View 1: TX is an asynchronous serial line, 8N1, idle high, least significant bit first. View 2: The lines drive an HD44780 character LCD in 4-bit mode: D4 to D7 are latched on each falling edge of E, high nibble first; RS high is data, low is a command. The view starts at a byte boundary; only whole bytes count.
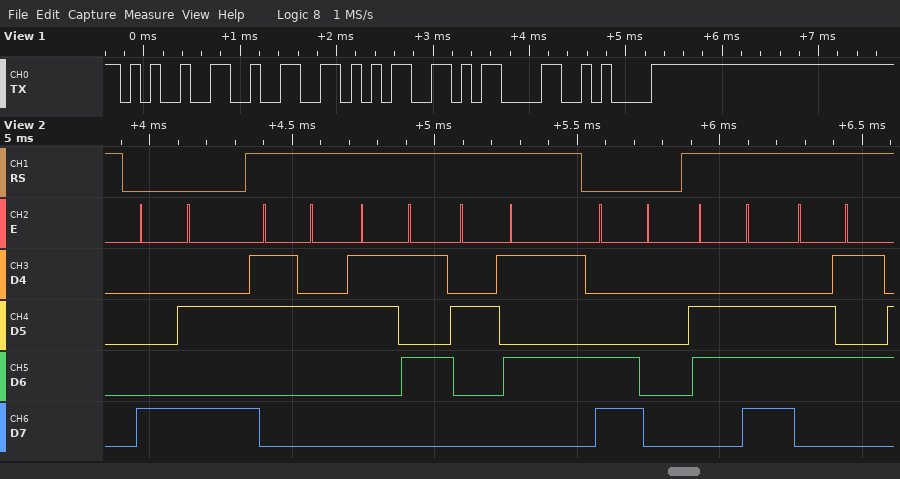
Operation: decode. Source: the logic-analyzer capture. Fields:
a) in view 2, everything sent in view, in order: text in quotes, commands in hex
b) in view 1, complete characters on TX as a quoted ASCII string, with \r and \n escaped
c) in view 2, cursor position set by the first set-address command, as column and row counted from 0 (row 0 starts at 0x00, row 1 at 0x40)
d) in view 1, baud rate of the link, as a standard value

0x8A "25%" 0xC0 "ne"
"%25\r\n"
column 10, row 0
9600 baud
